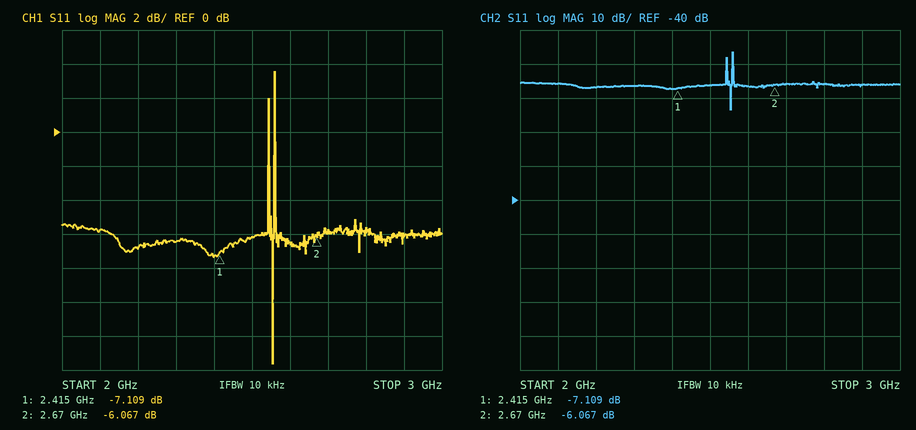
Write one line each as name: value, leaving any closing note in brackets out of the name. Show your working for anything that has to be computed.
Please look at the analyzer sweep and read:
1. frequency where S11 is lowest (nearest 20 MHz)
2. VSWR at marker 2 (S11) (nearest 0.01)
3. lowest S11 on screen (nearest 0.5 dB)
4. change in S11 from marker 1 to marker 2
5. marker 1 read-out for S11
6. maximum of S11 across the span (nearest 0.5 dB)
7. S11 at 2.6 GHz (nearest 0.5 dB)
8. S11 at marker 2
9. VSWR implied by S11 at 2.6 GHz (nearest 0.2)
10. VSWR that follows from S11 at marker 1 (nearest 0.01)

frequency where S11 is lowest: 2.56 GHz
VSWR at marker 2 (S11): (1 + 0.4973)/(1 − 0.4973) ≈ 2.98
lowest S11 on screen: -13.5 dB
change in S11 from marker 1 to marker 2: -6.067 − (-7.109) = 1.042 dB
marker 1 read-out for S11: -7.109 dB
maximum of S11 across the span: 3.5 dB
S11 at 2.6 GHz: -6.5 dB
S11 at marker 2: -6.067 dB
VSWR implied by S11 at 2.6 GHz: |Γ| = 10^(-6.5/20) = 0.4732; VSWR = (1 + 0.4732)/(1 − 0.4732) ≈ 2.8
VSWR that follows from S11 at marker 1: (1 + 0.4411)/(1 − 0.4411) ≈ 2.58
